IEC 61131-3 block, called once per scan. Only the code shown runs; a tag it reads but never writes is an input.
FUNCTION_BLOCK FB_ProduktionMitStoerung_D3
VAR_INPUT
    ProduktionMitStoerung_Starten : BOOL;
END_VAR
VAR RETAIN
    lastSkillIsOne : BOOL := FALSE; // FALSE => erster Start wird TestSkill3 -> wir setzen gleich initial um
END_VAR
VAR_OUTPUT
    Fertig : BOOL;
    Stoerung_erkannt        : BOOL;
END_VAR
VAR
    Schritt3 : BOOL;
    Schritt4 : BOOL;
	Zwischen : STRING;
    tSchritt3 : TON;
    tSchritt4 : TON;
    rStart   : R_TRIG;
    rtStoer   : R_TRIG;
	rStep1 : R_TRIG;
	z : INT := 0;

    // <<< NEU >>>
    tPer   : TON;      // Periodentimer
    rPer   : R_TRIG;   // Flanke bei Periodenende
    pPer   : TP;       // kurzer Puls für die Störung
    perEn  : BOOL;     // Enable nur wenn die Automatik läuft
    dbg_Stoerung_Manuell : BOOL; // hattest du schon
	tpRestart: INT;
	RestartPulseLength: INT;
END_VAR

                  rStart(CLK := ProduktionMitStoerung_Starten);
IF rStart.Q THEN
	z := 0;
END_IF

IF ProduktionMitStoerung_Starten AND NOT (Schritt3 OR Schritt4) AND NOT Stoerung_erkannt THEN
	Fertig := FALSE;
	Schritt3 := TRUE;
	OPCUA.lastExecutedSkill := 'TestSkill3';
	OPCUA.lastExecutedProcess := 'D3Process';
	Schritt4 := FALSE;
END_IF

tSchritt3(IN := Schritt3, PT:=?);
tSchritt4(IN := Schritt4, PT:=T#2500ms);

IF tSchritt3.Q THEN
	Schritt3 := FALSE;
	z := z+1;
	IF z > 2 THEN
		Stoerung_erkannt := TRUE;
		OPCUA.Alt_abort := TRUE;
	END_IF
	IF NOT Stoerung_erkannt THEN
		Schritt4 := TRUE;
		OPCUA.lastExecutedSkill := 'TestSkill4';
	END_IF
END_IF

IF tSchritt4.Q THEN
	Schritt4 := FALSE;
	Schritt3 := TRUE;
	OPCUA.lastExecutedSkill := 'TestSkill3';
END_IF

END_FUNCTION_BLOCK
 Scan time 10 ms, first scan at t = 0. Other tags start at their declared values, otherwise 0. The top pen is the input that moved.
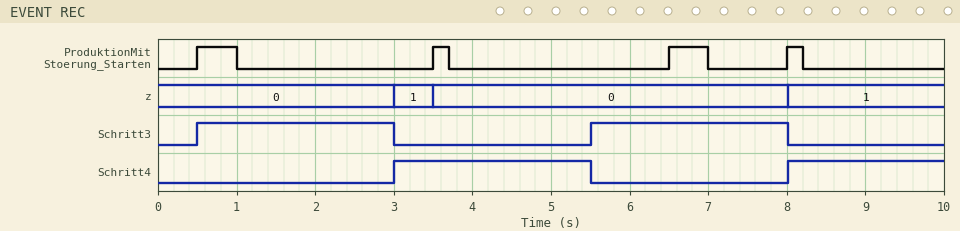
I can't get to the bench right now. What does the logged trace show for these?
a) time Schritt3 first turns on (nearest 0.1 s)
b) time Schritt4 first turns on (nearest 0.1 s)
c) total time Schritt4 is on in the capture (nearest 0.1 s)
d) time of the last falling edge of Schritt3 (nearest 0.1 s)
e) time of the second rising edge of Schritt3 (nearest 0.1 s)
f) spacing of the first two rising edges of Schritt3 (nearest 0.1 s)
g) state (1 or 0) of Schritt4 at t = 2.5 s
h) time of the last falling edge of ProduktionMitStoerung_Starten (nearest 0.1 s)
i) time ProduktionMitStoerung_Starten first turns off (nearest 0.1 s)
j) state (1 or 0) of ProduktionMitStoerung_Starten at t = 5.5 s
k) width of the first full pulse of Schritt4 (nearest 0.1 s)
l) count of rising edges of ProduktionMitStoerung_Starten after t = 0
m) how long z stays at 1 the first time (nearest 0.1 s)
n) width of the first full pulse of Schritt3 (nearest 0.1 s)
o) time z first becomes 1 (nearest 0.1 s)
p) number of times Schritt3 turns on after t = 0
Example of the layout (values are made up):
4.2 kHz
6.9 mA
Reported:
0.5 s
3.0 s
4.5 s
8.0 s
5.5 s
5.0 s
0
8.2 s
1.0 s
0
2.5 s
4
0.5 s
2.5 s
3.0 s
2
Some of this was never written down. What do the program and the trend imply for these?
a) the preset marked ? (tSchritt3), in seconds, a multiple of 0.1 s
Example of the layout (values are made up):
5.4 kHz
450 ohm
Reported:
2.5 s
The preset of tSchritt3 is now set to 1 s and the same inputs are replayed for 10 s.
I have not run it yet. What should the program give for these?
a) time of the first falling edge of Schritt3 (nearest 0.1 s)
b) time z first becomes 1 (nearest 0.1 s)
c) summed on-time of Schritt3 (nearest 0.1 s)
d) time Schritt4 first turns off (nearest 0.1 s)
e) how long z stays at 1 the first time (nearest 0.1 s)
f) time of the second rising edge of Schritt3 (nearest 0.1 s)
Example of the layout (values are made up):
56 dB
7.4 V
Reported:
1.5 s
1.5 s
3.0 s
4.0 s
2.0 s
4.0 s
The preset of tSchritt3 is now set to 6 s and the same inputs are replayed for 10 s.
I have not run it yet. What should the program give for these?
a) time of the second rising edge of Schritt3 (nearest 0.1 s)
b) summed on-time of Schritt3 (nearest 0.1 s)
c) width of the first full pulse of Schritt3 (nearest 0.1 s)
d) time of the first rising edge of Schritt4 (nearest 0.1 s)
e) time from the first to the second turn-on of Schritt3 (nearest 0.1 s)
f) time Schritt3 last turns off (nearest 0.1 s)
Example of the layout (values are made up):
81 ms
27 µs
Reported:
9.0 s
7.0 s
6.0 s
6.5 s
8.5 s
6.5 s
